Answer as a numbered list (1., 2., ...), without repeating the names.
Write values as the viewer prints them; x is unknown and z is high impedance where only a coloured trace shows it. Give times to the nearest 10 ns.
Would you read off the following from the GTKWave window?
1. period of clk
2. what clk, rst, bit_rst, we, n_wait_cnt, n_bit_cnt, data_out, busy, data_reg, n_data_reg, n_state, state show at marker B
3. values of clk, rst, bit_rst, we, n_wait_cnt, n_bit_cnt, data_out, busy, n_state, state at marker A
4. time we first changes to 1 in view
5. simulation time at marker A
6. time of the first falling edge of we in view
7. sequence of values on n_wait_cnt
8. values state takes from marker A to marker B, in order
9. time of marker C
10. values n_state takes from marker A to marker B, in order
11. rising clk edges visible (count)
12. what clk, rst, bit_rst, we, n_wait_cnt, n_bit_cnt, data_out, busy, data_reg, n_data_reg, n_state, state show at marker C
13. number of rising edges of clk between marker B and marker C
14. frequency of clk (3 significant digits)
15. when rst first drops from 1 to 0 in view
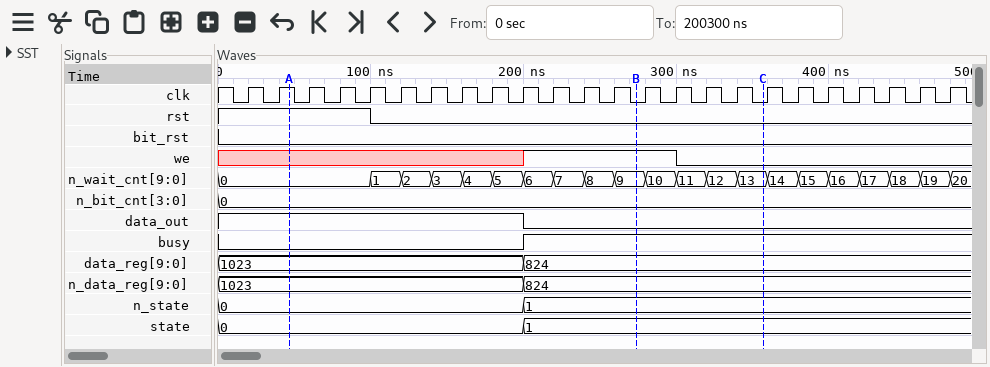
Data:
1. 20 ns
2. clk=0, rst=0, bit_rst=0, we=1, n_wait_cnt=9, n_bit_cnt=0, data_out=0, busy=1, data_reg=824, n_data_reg=824, n_state=1, state=1
3. clk=1, rst=1, bit_rst=0, we=x, n_wait_cnt=0, n_bit_cnt=0, data_out=1, busy=0, n_state=0, state=0
4. 200 ns
5. 50 ns
6. 300 ns
7. 0, 1, 2, 3, 4, 5, 6, 7, 8, 9, 10, 11, 12, 13, 14, 15, 16, 17, 18, 19, 20
8. 0, 1
9. 360 ns
10. 0, 1
11. 24
12. clk=0, rst=0, bit_rst=0, we=0, n_wait_cnt=13, n_bit_cnt=0, data_out=0, busy=1, data_reg=824, n_data_reg=824, n_state=1, state=1
13. 4
14. 50.0 MHz
15. 100 ns
